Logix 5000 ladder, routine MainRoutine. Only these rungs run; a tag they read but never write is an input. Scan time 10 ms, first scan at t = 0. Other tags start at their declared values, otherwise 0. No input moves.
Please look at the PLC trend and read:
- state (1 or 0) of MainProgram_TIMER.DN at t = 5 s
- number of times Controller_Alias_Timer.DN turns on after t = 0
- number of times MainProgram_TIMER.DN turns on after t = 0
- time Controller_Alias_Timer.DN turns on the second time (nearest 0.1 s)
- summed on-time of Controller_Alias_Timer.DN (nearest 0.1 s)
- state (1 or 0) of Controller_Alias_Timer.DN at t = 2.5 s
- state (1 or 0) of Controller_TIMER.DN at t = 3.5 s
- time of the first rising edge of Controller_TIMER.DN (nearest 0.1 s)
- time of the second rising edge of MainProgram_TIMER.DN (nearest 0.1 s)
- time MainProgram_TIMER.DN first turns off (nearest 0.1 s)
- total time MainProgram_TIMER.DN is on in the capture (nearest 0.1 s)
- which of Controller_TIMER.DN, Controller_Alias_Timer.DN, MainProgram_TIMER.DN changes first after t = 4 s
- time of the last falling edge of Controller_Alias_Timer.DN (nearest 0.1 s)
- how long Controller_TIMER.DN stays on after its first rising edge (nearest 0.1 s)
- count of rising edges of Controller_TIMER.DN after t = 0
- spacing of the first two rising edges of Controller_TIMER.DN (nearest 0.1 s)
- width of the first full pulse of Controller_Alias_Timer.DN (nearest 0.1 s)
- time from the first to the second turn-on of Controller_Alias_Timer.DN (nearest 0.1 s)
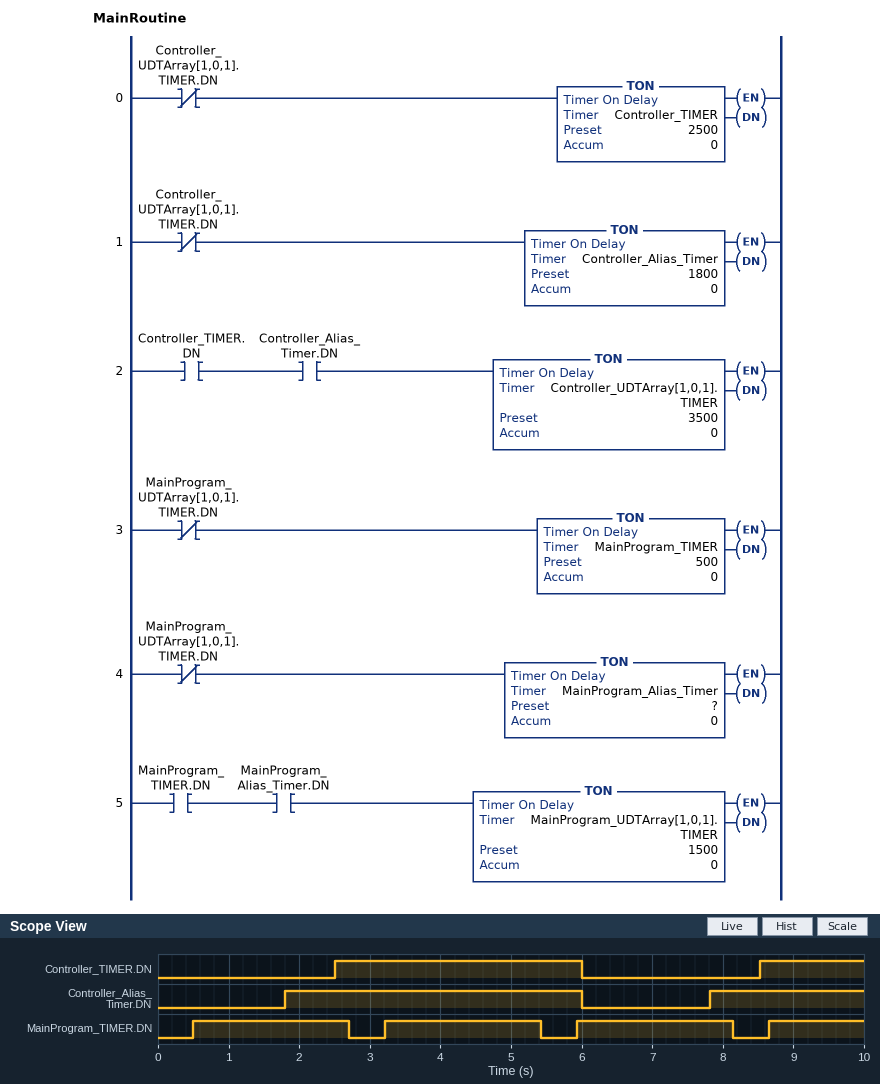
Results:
1
2
4
7.8 s
6.4 s
1
1
2.5 s
3.2 s
2.7 s
8.0 s
MainProgram_TIMER.DN
6.0 s
3.5 s
2
6.0 s
4.2 s
6.0 s
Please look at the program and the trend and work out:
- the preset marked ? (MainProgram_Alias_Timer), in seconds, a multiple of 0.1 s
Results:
1.2 s
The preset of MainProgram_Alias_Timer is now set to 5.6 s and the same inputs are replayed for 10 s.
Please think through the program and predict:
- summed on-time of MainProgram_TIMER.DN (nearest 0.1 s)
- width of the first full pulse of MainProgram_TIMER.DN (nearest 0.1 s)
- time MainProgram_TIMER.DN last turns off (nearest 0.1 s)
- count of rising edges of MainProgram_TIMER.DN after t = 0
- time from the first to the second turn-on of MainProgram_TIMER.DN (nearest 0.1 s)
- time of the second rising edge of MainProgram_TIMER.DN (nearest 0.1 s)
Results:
9.0 s
6.6 s
7.1 s
2
7.1 s
7.6 s
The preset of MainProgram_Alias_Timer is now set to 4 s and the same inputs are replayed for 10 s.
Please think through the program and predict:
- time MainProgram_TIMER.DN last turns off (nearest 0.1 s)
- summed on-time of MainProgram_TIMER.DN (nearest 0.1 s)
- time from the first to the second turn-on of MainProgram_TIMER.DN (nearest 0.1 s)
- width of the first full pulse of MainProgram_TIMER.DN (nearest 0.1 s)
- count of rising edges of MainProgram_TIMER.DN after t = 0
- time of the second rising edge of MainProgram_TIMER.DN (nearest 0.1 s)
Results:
5.5 s
9.0 s
5.5 s
5.0 s
2
6.0 s
